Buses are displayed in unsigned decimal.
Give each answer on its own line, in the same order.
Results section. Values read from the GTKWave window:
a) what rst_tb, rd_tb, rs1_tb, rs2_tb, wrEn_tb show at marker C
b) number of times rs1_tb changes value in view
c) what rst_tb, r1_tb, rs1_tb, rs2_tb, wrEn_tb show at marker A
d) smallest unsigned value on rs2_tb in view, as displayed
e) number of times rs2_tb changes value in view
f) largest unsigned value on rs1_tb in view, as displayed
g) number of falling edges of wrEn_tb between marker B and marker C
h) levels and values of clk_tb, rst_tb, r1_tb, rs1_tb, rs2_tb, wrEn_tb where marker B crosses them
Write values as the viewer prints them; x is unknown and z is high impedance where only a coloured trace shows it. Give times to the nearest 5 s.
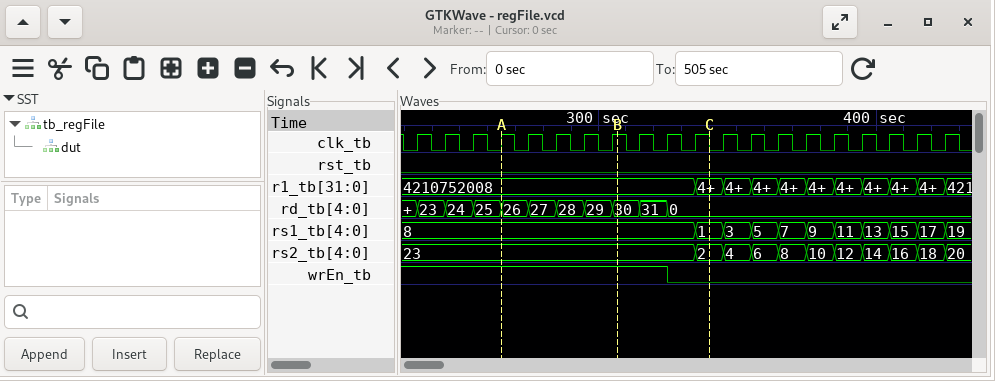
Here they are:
rst_tb=0, rd_tb=0, rs1_tb=1, rs2_tb=2, wrEn_tb=0
10
rst_tb=0, r1_tb=4210752008, rs1_tb=8, rs2_tb=23, wrEn_tb=1
2
10
19
1
clk_tb=1, rst_tb=0, r1_tb=4210752008, rs1_tb=8, rs2_tb=23, wrEn_tb=1
